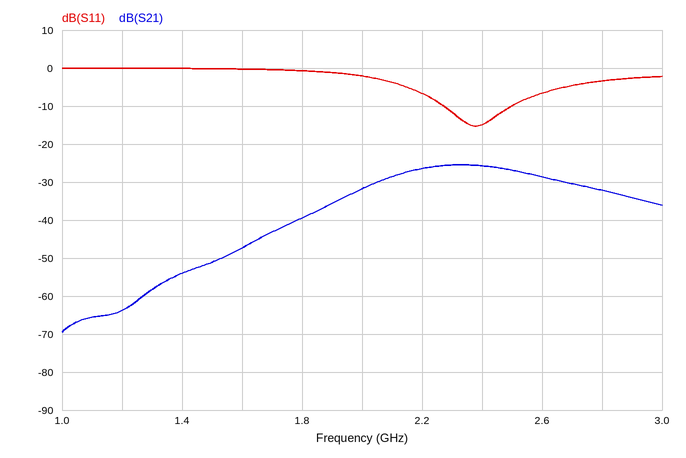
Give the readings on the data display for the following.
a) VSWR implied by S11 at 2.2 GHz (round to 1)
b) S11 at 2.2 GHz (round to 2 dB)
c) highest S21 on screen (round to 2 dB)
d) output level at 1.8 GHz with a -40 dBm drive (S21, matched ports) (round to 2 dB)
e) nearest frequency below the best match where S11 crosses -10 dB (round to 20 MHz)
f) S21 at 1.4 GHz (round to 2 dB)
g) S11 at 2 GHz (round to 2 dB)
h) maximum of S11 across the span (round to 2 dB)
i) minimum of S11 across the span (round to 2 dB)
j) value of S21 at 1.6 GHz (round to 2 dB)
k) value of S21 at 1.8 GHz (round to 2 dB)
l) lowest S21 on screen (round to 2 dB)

3
-6 dB
-26 dB
-80 dBm
2.28 GHz
-54 dB
-2 dB
0 dB
-16 dB
-48 dB
-40 dB
-70 dB
